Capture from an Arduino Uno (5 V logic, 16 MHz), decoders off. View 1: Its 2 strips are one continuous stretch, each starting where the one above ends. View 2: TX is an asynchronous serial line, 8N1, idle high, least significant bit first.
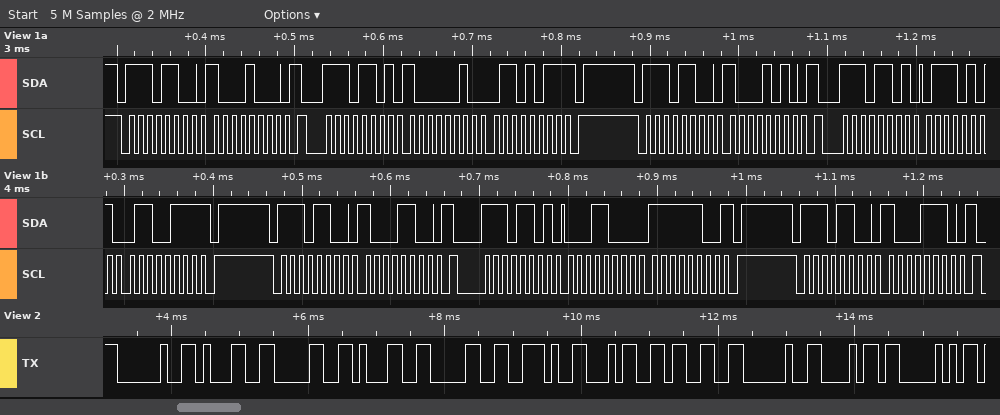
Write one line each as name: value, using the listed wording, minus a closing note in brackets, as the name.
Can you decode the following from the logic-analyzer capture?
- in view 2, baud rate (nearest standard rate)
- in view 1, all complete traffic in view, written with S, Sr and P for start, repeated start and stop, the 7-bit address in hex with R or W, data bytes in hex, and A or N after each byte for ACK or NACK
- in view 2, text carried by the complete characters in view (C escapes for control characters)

in view 2, baud rate: 9600 baud
in view 1, all complete traffic in view, written with S, Sr and P for start, repeated start and stop, the 7-bit address in hex with R or W, data bytes in hex, and A or N after each byte for ACK or NACK: S 76W A 88 A Sr 76R A 82 A 6B N P S 76W A 8A A Sr 76R A 75 A 67 N P S 76W A 8C A Sr 76R A 18 A FC N P S 76W A 8E A
in view 2, text carried by the complete characters in view: " 1010.43 hP"
